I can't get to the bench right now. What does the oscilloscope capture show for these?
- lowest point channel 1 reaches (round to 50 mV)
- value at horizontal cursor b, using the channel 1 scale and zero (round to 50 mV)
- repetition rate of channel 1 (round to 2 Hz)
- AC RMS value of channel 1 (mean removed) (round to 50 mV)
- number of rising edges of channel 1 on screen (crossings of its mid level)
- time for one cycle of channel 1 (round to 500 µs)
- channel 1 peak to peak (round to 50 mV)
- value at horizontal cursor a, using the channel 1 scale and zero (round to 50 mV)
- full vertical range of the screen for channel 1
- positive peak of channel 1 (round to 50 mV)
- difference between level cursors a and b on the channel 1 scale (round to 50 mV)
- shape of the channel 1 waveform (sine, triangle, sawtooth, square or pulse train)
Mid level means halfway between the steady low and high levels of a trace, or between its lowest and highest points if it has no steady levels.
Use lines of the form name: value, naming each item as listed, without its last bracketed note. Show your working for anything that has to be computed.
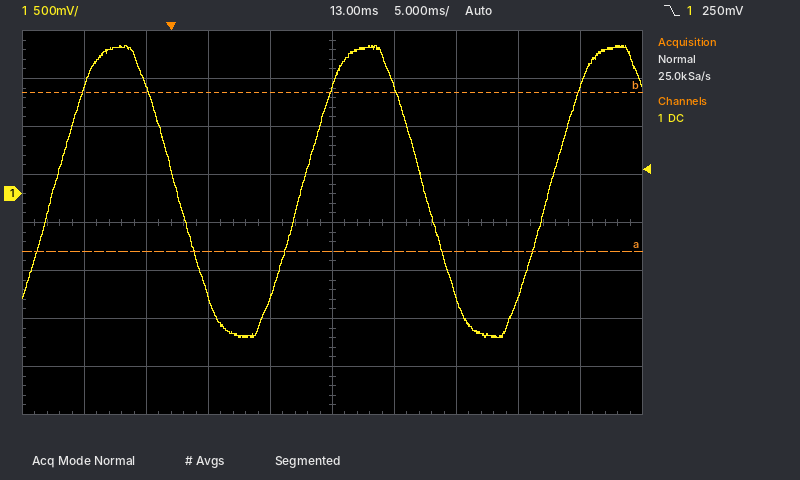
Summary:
lowest point channel 1 reaches: -1.50 V
value at horizontal cursor b, using the channel 1 scale and zero: 1.05 V
repetition rate of channel 1: 1 / 20.0 ms ≈ 50 Hz
AC RMS value of channel 1 (mean removed): 3.05 V / (2√2) ≈ 1.08 V, so 1.10 V to the nearest 50 mV
number of rising edges of channel 1 on screen: 3
time for one cycle of channel 1: 20.0 ms
channel 1 peak to peak: 1.55 V − (-1.50 V) = 3.05 V
value at horizontal cursor a, using the channel 1 scale and zero: -600 mV
full vertical range of the screen for channel 1: 4 V
positive peak of channel 1: 1.55 V
difference between level cursors a and b on the channel 1 scale: 1.65 V
shape of the channel 1 waveform: sine
